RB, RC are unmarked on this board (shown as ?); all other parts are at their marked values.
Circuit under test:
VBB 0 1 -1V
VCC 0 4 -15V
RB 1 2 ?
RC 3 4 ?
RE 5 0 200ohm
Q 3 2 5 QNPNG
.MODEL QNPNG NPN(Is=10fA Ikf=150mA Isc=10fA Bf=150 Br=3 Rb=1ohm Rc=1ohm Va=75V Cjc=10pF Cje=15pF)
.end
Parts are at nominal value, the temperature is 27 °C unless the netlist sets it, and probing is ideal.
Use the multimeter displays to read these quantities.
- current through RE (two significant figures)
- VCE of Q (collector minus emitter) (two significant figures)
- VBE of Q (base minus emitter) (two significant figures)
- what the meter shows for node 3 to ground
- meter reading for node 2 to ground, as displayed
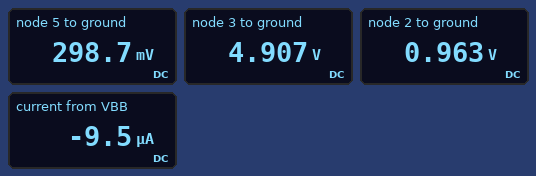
1.5 mA
4.6 V
660 mV
4.907 V
0.963 V
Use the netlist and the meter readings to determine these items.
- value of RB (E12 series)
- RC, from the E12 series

3.9 kΩ
6.8 kΩ
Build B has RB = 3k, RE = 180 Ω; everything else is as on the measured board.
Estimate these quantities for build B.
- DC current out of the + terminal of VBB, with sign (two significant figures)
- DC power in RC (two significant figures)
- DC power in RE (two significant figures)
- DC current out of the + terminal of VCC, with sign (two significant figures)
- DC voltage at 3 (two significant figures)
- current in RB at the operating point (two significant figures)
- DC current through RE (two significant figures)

-11 µA
19 mW
500 µW
-1.7 mA
3.7 V
11 µA
1.7 mA
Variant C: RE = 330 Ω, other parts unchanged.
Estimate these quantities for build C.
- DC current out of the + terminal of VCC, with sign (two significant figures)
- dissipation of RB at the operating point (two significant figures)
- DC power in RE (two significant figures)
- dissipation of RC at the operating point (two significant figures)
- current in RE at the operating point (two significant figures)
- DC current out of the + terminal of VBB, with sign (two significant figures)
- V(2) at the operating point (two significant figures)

-980 µA
140 nW
320 µW
6.5 mW
980 µA
-6.0 µA
980 mV
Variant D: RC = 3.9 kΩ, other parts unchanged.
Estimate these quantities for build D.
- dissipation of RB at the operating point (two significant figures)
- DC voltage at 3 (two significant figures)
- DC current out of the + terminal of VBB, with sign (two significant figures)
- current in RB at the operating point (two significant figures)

320 nW
9.2 V
-9.1 µA
9.1 µA
